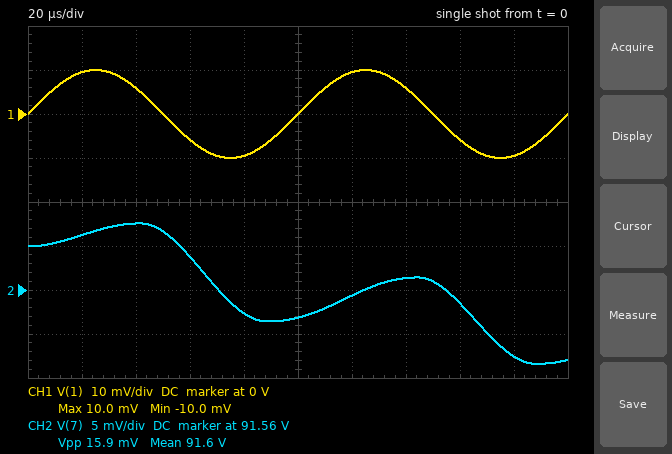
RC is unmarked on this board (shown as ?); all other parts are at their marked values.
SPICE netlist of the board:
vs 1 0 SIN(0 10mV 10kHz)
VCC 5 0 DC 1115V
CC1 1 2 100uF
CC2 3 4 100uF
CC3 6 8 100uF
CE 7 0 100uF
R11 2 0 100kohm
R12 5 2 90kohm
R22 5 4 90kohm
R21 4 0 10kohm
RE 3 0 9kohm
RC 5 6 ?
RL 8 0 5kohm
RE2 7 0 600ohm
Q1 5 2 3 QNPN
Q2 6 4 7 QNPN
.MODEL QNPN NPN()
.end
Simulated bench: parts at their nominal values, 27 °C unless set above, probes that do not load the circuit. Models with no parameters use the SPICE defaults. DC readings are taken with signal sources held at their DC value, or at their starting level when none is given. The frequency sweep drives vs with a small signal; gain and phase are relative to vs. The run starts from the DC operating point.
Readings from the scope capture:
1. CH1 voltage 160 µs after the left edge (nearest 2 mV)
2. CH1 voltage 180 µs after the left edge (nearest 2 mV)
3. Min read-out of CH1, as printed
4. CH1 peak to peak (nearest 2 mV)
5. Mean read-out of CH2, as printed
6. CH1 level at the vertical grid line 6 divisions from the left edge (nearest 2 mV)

-6 mV
-10 mV
-10.0 mV
20 mV
91.6 V
10 mV
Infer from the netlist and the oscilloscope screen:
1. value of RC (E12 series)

6.8 kΩ
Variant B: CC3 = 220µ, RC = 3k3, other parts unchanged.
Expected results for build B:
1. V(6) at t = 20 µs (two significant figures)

530 V
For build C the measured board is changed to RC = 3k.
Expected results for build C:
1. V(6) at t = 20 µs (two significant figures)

580 V
